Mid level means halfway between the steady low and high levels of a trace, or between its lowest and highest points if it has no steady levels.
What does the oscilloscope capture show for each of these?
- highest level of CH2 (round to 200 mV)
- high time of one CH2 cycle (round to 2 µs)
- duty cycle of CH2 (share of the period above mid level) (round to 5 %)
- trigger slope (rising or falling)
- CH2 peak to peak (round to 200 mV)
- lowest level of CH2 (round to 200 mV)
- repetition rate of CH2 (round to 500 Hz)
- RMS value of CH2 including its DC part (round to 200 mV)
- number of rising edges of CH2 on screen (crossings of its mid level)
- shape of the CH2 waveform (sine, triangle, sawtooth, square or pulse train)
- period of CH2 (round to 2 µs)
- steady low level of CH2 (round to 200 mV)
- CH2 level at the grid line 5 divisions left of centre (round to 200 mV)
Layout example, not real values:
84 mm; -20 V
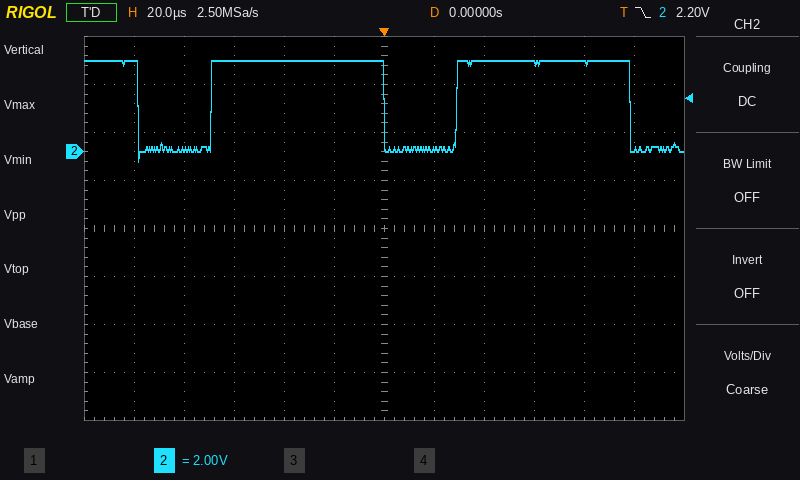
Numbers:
3.8 V; 70 µs; 70 %; falling; 4.2 V; -400 mV; 10.0 kHz; 3.2 V; 2; pulse train; 98 µs; 0.0 V; 3.8 V
